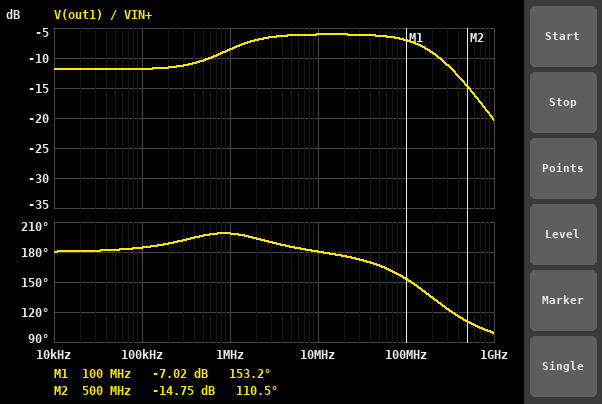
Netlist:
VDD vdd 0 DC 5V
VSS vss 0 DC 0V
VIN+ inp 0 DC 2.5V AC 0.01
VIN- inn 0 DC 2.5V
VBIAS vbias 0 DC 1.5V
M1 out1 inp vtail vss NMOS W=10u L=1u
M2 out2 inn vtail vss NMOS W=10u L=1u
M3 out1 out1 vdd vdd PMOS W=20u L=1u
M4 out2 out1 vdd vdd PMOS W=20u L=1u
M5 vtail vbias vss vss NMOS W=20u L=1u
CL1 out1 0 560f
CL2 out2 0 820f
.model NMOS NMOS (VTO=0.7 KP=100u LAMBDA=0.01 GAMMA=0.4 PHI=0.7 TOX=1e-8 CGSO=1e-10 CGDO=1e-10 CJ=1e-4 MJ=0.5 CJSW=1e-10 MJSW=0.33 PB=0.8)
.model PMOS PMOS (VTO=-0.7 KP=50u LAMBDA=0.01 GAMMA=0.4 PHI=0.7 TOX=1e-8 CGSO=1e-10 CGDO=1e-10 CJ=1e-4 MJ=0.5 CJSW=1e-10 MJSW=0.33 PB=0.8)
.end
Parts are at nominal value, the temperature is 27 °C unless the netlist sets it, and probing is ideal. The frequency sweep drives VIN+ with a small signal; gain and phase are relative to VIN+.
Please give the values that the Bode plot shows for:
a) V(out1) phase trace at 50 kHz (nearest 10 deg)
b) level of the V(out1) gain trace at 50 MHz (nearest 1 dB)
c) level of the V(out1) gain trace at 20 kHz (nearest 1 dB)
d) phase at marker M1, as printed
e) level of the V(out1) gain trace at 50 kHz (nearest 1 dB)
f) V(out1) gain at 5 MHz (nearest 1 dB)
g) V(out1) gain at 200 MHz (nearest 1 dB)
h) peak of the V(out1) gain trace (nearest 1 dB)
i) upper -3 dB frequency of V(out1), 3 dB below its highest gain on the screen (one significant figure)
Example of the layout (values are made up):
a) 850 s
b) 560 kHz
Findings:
a) 180 deg
b) -6 dB
c) -12 dB
d) 153.2 deg
e) -12 dB
f) -6 dB
g) -9 dB
h) -6 dB
i) 200 MHz
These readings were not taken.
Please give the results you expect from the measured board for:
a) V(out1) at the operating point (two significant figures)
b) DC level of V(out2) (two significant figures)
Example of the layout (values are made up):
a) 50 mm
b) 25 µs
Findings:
a) 3.5 V
b) 3.5 V
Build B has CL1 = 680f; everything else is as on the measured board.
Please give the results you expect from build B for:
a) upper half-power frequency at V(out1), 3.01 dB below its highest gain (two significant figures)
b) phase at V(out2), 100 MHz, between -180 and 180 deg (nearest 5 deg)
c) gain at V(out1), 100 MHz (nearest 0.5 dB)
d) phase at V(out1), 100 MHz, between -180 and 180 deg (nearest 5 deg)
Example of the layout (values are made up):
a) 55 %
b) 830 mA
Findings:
a) 170 MHz
b) -105 deg
c) -7.5 dB
d) 150 deg
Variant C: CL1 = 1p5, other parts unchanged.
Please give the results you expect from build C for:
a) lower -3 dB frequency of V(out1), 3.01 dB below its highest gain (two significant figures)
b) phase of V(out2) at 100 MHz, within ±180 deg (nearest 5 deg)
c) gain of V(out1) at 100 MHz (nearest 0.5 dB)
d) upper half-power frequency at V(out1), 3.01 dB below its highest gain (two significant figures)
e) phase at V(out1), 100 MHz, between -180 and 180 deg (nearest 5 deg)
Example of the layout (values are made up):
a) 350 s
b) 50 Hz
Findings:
a) 820 kHz
b) -110 deg
c) -10.0 dB
d) 83 MHz
e) 130 deg
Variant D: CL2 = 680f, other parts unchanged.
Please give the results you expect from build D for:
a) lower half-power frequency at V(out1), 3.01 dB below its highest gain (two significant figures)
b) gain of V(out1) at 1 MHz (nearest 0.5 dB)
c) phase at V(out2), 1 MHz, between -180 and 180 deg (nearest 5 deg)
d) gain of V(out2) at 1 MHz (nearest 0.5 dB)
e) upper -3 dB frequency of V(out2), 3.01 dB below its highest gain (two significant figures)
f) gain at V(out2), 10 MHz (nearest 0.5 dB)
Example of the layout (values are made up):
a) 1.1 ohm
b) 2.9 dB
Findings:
a) 1.0 MHz
b) -9.0 dB
c) -35 deg
d) 40.5 dB
e) 1.5 MHz
f) 25.5 dB
